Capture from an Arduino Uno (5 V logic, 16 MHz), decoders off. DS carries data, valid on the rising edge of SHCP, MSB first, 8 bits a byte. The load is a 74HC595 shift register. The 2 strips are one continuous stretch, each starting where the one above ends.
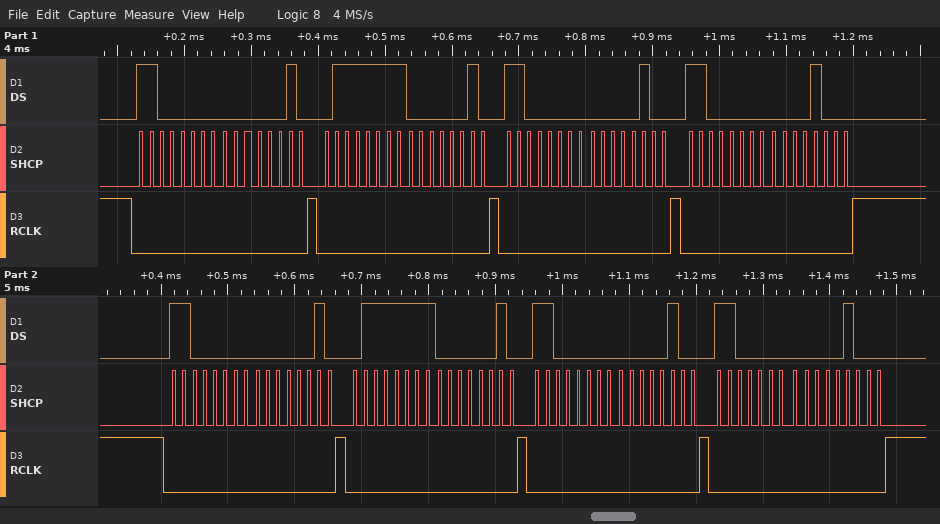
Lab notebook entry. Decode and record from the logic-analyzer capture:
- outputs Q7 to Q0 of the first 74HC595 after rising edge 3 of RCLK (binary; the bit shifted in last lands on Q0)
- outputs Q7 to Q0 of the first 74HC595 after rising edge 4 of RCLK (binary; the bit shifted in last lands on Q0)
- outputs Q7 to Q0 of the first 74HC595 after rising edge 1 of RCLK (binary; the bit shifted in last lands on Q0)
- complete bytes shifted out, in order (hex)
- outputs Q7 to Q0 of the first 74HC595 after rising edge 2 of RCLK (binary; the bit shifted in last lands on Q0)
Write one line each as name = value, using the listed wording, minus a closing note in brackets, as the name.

outputs Q7 to Q0 of the first 74HC595 after rising edge 3 of RCLK = 00000100
outputs Q7 to Q0 of the first 74HC595 after rising edge 4 of RCLK = 00001000
outputs Q7 to Q0 of the first 74HC595 after rising edge 1 of RCLK = 00000010
complete bytes shifted out, in order = C0 02 7F 02 C0 04 C0 08 C0 02 7F 02 C0 04 C0 08
outputs Q7 to Q0 of the first 74HC595 after rising edge 2 of RCLK = 00000010
